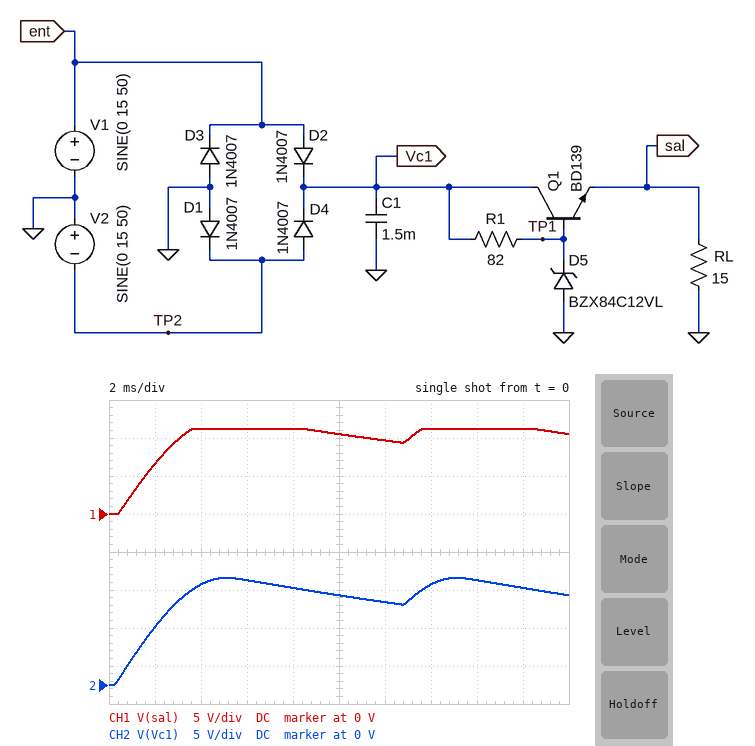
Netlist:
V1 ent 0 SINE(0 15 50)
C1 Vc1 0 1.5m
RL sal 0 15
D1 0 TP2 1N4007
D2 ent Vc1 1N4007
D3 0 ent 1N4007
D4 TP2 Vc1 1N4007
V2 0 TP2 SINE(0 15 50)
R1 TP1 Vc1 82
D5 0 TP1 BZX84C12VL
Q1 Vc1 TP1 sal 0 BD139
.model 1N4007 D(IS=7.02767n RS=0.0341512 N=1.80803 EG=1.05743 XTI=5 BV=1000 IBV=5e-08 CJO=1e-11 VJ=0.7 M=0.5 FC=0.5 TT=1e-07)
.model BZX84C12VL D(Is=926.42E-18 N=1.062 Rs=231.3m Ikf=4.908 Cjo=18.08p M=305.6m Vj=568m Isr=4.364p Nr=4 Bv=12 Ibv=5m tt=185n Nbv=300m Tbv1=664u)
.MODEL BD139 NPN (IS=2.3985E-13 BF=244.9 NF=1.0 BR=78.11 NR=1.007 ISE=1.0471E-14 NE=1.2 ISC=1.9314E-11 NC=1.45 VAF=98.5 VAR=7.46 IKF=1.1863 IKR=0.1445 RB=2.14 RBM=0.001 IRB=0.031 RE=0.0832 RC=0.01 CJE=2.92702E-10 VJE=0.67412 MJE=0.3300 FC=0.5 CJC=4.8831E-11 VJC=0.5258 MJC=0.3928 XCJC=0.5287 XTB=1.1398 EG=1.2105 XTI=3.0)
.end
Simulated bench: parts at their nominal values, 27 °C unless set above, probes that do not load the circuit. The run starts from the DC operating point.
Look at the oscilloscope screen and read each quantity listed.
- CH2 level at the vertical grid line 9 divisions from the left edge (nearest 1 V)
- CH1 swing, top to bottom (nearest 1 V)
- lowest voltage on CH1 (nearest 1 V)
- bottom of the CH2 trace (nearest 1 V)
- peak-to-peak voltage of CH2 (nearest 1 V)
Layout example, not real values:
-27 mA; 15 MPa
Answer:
13 V; 11 V; 0 V; 0 V; 14 V
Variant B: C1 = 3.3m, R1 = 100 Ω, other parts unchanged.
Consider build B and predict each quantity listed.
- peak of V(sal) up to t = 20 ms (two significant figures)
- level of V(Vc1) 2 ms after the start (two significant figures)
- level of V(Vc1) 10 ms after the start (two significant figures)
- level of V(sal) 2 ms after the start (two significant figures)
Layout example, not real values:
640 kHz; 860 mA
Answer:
11 V; 7.4 V; 13 V; 6.3 V
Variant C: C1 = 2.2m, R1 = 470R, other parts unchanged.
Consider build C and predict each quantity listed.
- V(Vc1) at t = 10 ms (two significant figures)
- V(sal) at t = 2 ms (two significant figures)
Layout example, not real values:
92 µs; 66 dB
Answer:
13 V; 5.6 V
